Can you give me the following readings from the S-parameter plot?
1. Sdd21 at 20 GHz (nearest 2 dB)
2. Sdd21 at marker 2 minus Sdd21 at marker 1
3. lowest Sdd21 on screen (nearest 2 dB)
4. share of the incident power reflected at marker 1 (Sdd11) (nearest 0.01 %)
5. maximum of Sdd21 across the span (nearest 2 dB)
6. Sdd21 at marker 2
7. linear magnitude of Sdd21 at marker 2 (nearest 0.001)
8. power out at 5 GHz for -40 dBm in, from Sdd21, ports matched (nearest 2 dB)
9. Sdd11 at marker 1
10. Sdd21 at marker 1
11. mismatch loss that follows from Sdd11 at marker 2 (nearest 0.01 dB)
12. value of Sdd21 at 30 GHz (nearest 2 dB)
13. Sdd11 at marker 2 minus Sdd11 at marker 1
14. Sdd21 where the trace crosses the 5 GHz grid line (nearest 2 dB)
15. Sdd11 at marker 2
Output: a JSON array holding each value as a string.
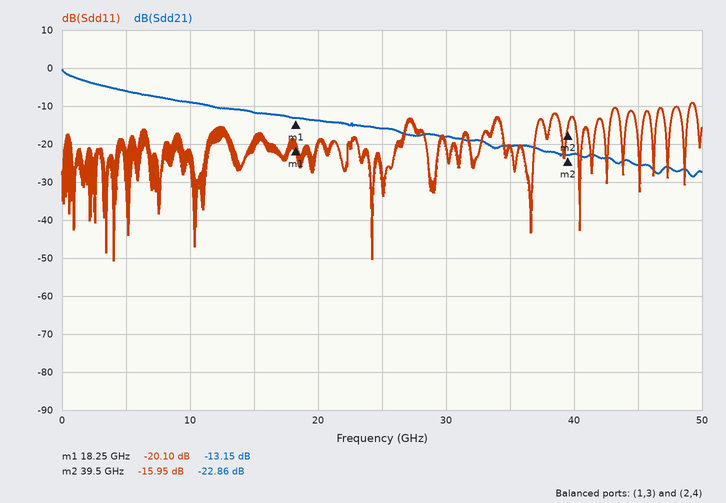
["-14 dB", "-9.71 dB", "-28 dB", "0.98 %", "0 dB", "-22.86 dB", "0.072", "-46 dBm", "-20.10 dB", "-13.15 dB", "0.11 dB", "-18 dB", "4.15 dB", "-6 dB", "-15.95 dB"]
